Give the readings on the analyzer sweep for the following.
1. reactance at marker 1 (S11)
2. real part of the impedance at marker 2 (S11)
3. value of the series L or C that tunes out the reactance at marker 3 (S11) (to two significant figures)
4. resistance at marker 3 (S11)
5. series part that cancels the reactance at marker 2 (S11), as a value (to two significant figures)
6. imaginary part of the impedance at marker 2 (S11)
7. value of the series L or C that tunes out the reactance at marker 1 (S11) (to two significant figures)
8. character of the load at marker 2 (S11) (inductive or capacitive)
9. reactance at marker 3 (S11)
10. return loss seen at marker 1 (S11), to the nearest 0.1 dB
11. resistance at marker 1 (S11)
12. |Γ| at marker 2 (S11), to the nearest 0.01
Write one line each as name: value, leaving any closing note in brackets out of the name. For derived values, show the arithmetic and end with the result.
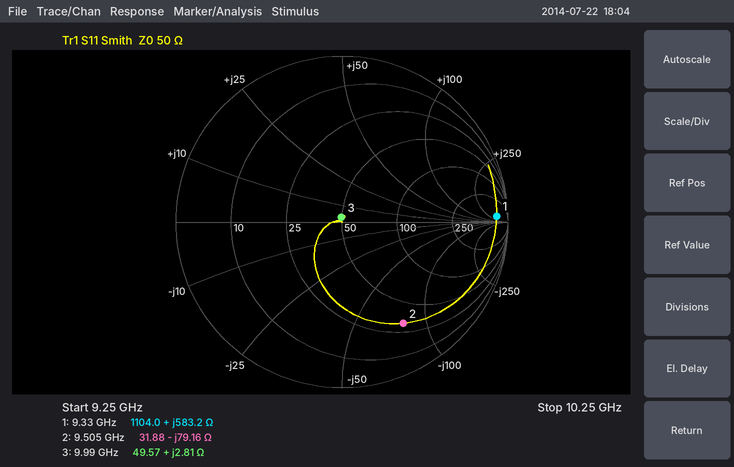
reactance at marker 1: +583.2 Ω
real part of the impedance at marker 2: 31.88 Ω
value of the series L or C that tunes out the reactance at marker 3 (S11): C = 1/(2π × 9.99 GHz × 2.81 Ω) ≈ 5.7 pF
resistance at marker 3: 49.57 Ω
series part that cancels the reactance at marker 2 (S11), as a value: L = 79.16 Ω/(2π × 9.505 GHz) ≈ 1.3 nH
imaginary part of the impedance at marker 2: -79.16 Ω
value of the series L or C that tunes out the reactance at marker 1 (S11): C = 1/(2π × 9.33 GHz × 583.2 Ω) ≈ 29 fF
character of the load at marker 2 (S11): capacitive
reactance at marker 3: +2.81 Ω
return loss seen at marker 1 (S11), to the nearest 0.1 dB: 0.6 dB
resistance at marker 1: 1104.0 Ω
|Γ| at marker 2 (S11), to the nearest 0.01: 0.71
